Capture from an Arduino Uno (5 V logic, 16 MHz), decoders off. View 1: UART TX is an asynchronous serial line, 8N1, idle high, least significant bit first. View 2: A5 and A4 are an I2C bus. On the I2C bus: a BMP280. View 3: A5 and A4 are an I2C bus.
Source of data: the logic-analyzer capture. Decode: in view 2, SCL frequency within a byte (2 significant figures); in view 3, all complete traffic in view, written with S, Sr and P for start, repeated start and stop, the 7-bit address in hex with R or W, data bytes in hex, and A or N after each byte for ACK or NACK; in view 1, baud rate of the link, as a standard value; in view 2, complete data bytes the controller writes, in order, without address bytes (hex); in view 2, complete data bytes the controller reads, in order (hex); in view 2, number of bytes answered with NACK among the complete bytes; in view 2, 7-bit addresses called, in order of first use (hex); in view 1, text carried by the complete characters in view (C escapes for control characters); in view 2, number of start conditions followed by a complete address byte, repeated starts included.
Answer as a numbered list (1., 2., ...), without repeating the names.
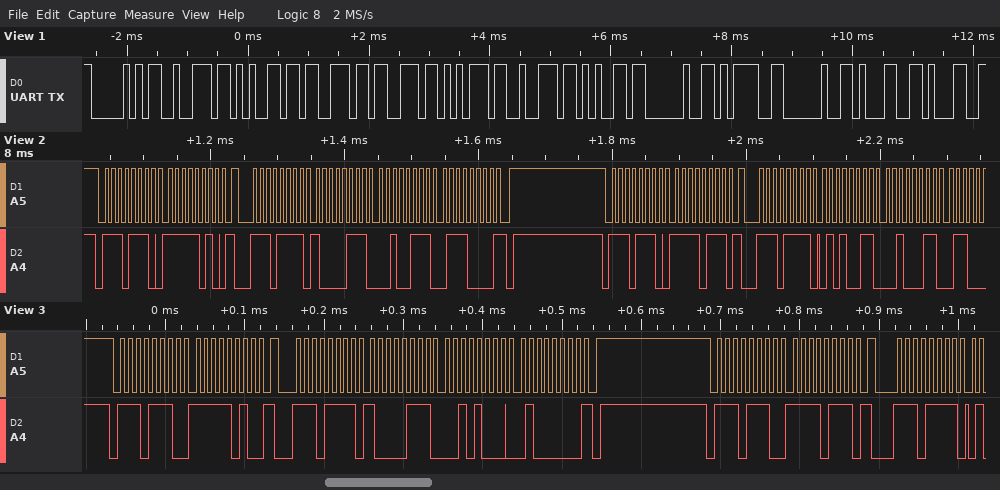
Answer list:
1. 100 kHz
2. S 77W A FA A Sr 77R A 87 A 28 A 40 N P S 77W A F7 A Sr 77R A
3. 9600 baud
4. FA F7
5. 87 27 70 53 23
6. 1
7. 0x77
8. "Pressure = 11"
9. 4
